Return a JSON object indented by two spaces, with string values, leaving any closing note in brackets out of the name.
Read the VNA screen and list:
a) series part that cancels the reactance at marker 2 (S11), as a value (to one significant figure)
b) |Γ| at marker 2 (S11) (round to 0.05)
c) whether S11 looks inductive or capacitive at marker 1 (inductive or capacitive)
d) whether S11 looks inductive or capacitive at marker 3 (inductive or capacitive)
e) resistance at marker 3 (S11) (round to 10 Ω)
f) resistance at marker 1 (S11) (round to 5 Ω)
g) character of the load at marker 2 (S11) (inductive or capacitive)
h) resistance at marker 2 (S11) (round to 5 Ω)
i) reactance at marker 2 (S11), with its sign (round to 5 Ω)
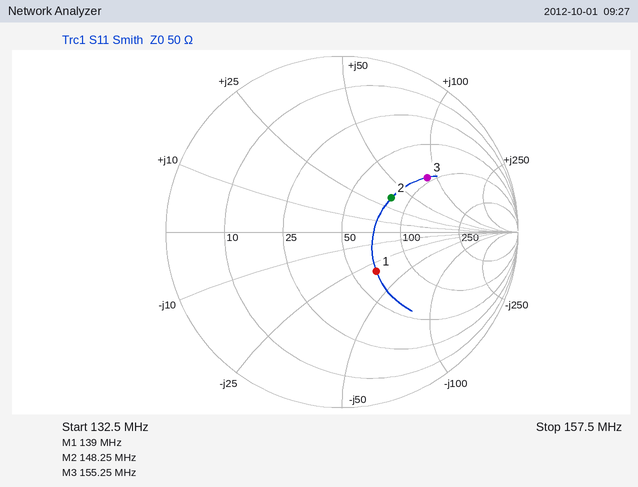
{
  "series part that cancels the reactance at marker 2 (S11), as a value": "30 pF",
  "|Γ| at marker 2 (S11)": "0.35",
  "whether S11 looks inductive or capacitive at marker 1": "capacitive",
  "whether S11 looks inductive or capacitive at marker 3": "inductive",
  "resistance at marker 3 (S11)": "90 Ω",
  "resistance at marker 1 (S11)": "65 Ω",
  "character of the load at marker 2 (S11)": "inductive",
  "resistance at marker 2 (S11)": "80 Ω",
  "reactance at marker 2 (S11), with its sign": "+35 Ω"
}
